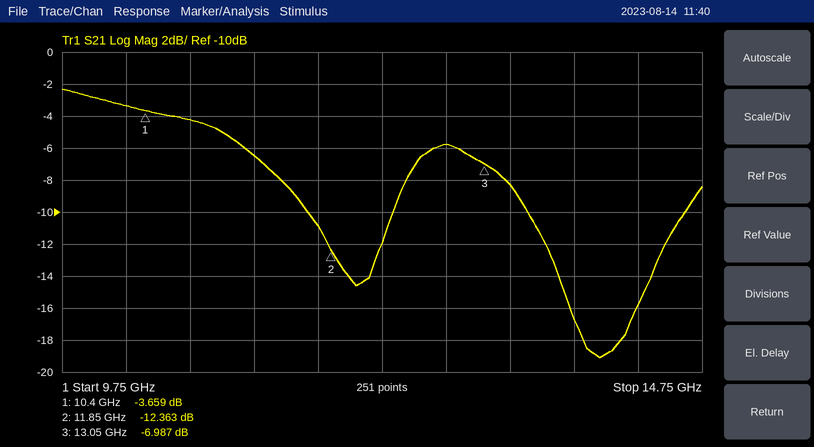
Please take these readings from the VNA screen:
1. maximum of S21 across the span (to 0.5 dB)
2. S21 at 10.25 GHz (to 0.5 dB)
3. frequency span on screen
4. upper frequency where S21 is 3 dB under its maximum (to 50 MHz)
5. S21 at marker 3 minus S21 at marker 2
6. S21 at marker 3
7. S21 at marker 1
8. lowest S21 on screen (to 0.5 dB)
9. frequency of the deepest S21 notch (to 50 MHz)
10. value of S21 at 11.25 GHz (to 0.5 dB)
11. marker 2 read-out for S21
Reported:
-2.5 dB
-3.5 dB
5 GHz
11.05 GHz
5.376 dB
-6.987 dB
-3.659 dB
-19.0 dB
13.95 GHz
-6.5 dB
-12.363 dB
